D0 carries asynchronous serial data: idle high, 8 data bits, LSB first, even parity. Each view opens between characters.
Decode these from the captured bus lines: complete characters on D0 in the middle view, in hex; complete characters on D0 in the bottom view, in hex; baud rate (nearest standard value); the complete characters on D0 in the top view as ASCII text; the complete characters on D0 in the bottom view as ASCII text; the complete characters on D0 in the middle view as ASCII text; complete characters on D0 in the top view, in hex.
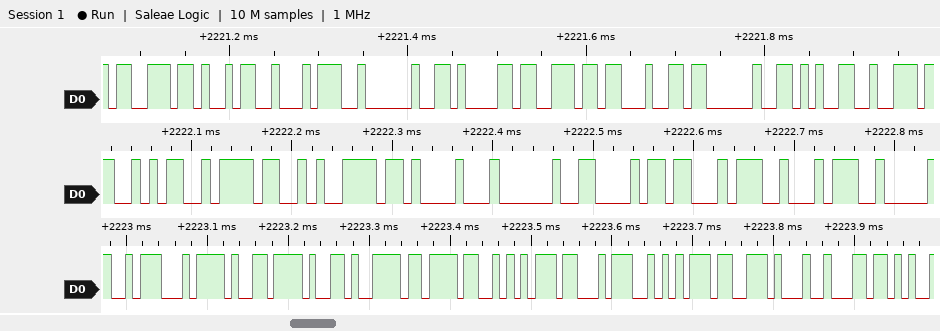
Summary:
6A, 6F, 79, 21, 20, 68, 74, 74
3A, 2F, 2F, 79, 6F, 75, 74, 75, 2E, 62
115200 baud
"sit and e"
"://youtu.b"
"joy! htt"
73, 69, 74, 20, 61, 6E, 64, 20, 65
